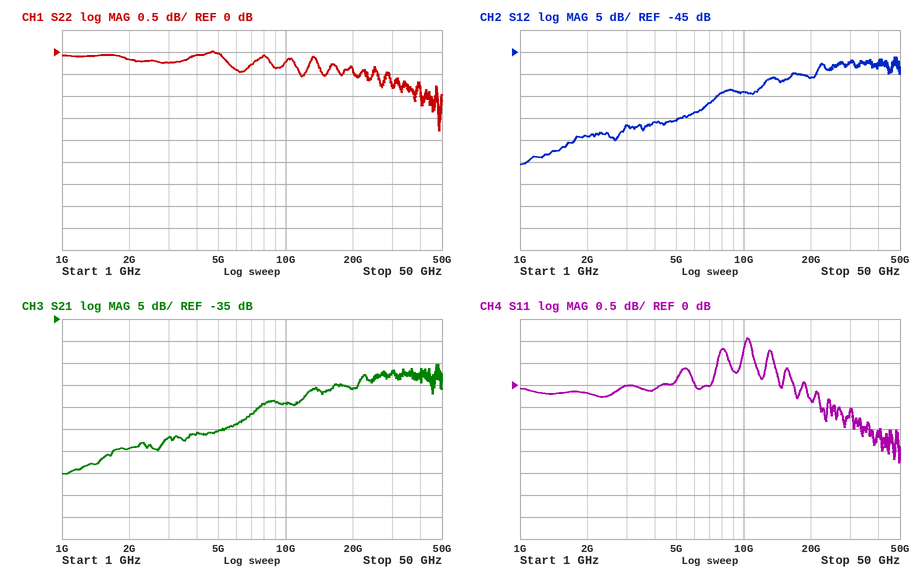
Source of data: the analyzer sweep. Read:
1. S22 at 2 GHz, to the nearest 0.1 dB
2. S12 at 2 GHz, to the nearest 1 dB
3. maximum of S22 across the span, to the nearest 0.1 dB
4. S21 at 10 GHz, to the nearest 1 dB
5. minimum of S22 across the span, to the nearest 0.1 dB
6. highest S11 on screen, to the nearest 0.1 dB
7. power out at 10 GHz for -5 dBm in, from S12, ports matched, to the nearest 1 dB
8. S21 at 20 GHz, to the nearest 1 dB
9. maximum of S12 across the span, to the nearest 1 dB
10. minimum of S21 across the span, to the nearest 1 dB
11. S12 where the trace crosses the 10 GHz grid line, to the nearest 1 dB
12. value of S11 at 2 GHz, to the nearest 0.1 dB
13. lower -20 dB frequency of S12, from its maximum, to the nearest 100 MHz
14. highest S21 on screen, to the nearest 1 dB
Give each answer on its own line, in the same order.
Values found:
-0.2 dB
-64 dB
0.0 dB
-54 dB
-1.8 dB
1.1 dB
-59 dBm
-51 dB
-46 dB
-70 dB
-54 dB
-0.2 dB
1.6 GHz
-45 dB
